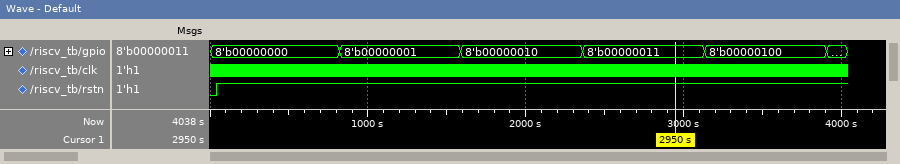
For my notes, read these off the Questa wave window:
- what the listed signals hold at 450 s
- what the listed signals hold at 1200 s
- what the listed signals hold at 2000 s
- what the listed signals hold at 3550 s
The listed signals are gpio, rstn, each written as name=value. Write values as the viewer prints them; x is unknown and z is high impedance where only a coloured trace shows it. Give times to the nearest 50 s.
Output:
gpio=8'b00000000, rstn=1
gpio=8'b00000001, rstn=1
gpio=8'b00000010, rstn=1
gpio=8'b00000100, rstn=1
